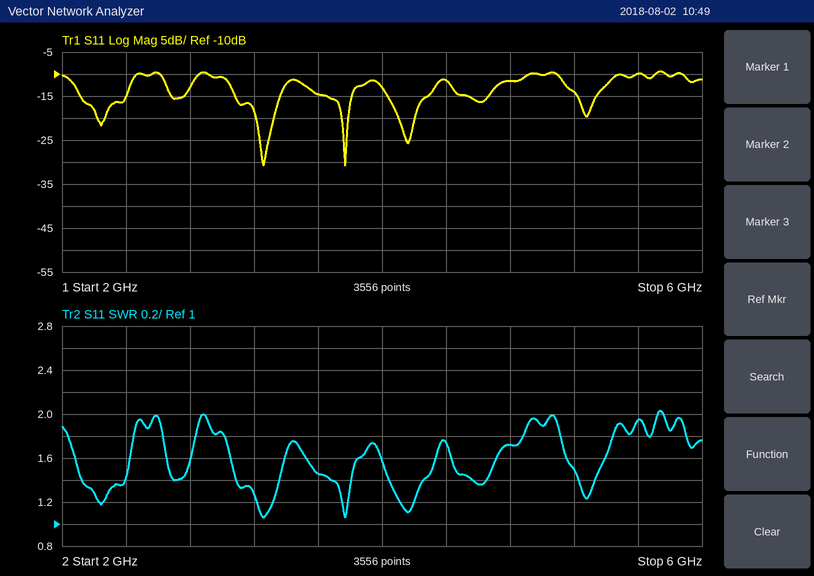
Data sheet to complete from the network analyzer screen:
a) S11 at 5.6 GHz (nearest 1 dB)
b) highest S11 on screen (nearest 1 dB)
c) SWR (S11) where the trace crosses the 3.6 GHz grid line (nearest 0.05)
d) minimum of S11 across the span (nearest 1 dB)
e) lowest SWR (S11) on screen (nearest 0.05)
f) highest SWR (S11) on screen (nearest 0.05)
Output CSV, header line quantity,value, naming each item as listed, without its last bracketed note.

quantity,value
S11 at 5.6 GHz,-10 dB
highest S11 on screen,-9 dB
SWR (S11) where the trace crosses the 3.6 GHz grid line,1.45
minimum of S11 across the span,-31 dB
lowest SWR (S11) on screen,1.05
highest SWR (S11) on screen,2.05
